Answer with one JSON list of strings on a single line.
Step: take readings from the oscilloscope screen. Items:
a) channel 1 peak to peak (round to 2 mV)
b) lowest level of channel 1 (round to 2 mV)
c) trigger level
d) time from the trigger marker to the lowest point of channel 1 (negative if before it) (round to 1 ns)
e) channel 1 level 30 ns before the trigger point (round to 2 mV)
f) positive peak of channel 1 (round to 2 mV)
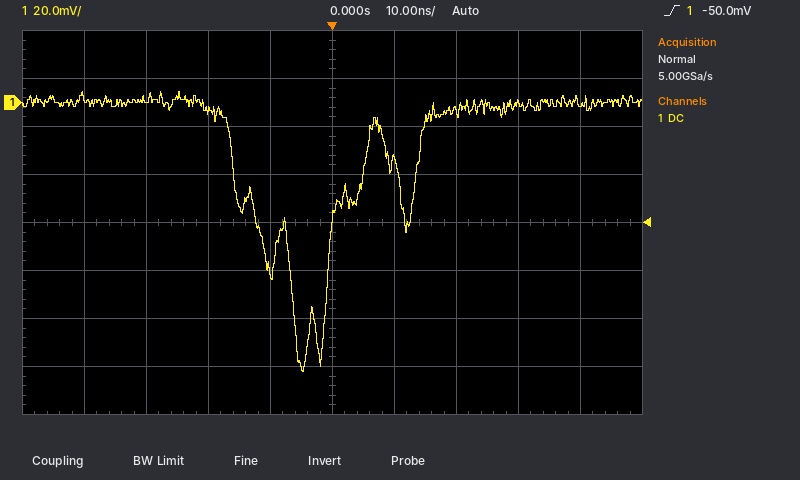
["116 mV", "-112 mV", "-50.0 mV", "-5 ns", "2 mV", "4 mV"]
